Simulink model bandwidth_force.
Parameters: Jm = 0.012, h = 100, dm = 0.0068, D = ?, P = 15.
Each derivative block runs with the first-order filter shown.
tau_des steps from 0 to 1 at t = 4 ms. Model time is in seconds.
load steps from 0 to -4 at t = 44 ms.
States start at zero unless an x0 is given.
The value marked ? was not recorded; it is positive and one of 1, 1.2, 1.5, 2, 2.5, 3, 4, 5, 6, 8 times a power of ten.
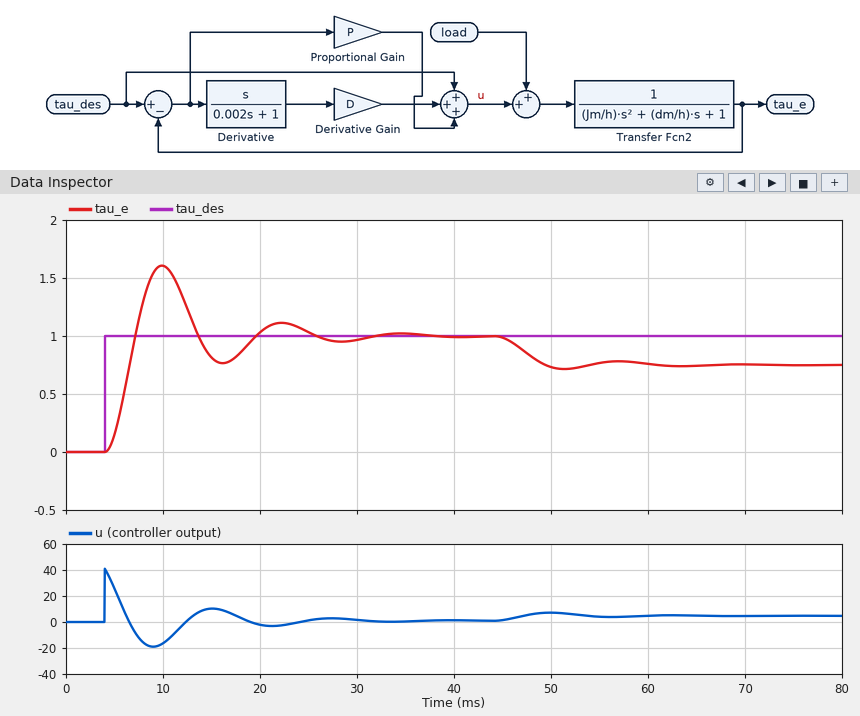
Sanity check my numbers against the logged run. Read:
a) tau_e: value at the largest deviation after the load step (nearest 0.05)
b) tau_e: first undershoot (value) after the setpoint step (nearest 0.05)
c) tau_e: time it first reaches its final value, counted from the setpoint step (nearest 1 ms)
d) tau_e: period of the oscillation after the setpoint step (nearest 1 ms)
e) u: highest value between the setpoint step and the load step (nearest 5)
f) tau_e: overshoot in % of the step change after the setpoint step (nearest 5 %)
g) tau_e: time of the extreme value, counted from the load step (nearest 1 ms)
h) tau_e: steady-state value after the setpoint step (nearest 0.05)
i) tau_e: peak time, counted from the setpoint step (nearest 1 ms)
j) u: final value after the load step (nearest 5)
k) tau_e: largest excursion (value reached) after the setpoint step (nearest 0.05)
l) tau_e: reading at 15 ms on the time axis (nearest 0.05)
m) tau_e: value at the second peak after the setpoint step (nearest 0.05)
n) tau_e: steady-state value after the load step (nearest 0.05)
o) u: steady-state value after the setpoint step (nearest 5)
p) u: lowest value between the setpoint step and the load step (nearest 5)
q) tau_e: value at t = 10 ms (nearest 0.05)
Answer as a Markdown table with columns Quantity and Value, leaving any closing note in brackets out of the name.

| Quantity | Value |
|---|---|
| tau_e: value at the largest deviation after the load step | 0.70 |
| tau_e: first undershoot (value) after the setpoint step | 0.75 |
| tau_e: time it first reaches its final value, counted from the setpoint step | 3 ms |
| tau_e: period of the oscillation after the setpoint step | 12 ms |
| u: highest value between the setpoint step and the load step | 40 |
| tau_e: overshoot in % of the step change after the setpoint step | 60 % |
| tau_e: time of the extreme value, counted from the load step | 7 ms |
| tau_e: steady-state value after the setpoint step | 1.00 |
| tau_e: peak time, counted from the setpoint step | 6 ms |
| u: final value after the load step | 5 |
| tau_e: largest excursion (value reached) after the setpoint step | 1.60 |
| tau_e: reading at 15 ms on the time axis | 0.80 |
| tau_e: value at the second peak after the setpoint step | 1.10 |
| tau_e: steady-state value after the load step | 0.75 |
| u: steady-state value after the setpoint step | 0 |
| u: lowest value between the setpoint step and the load step | -20 |
| tau_e: value at t = 10 ms | 1.60 |
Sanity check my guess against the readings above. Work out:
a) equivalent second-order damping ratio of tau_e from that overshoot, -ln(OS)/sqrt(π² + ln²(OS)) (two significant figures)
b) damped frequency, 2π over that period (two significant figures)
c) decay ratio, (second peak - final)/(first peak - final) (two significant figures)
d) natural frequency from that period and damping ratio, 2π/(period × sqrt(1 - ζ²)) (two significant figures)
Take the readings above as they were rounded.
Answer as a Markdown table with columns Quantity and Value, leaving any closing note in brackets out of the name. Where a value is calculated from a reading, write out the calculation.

| Quantity | Value |
|---|---|
| equivalent second-order damping ratio of tau_e from that overshoot, -ln(OS)/sqrt(π² + ln²(OS)) | ln(0.6) = -0.511; 0.511 / sqrt(9.870 + 0.261) = 0.16 |
| damped frequency, 2π over that period | 2π / 12 = 0.52 rad/ms |
| decay ratio, (second peak - final)/(first peak - final) | (1.1 - 1) / (1.6 - 1) = 0.17 |
| natural frequency from that period and damping ratio, 2π/(period × sqrt(1 - ζ²)) | 2π / (12 × sqrt(1 - 0.16²)) = 0.53 rad/ms |
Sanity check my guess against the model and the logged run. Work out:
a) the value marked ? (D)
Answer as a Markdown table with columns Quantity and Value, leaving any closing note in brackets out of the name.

| Quantity | Value |
|---|---|
| the value marked ? | 0.05 |
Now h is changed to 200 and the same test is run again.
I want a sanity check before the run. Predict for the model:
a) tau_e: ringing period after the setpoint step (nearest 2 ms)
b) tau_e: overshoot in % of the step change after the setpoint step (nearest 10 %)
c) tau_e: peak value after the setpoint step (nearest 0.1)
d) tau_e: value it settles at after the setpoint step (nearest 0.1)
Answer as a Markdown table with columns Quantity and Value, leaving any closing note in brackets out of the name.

| Quantity | Value |
|---|---|
| tau_e: ringing period after the setpoint step | 8 ms |
| tau_e: overshoot in % of the step change after the setpoint step | 70 % |
| tau_e: peak value after the setpoint step | 1.7 |
| tau_e: value it settles at after the setpoint step | 1.0 |
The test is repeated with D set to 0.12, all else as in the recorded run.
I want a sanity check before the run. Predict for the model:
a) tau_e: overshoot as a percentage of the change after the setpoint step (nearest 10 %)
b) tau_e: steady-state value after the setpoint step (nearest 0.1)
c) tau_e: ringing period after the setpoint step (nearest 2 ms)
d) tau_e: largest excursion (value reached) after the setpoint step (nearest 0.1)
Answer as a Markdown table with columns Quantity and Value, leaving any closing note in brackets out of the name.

| Quantity | Value |
|---|---|
| tau_e: overshoot as a percentage of the change after the setpoint step | 50 % |
| tau_e: steady-state value after the setpoint step | 1.0 |
| tau_e: ringing period after the setpoint step | 8 ms |
| tau_e: largest excursion (value reached) after the setpoint step | 1.5 |
